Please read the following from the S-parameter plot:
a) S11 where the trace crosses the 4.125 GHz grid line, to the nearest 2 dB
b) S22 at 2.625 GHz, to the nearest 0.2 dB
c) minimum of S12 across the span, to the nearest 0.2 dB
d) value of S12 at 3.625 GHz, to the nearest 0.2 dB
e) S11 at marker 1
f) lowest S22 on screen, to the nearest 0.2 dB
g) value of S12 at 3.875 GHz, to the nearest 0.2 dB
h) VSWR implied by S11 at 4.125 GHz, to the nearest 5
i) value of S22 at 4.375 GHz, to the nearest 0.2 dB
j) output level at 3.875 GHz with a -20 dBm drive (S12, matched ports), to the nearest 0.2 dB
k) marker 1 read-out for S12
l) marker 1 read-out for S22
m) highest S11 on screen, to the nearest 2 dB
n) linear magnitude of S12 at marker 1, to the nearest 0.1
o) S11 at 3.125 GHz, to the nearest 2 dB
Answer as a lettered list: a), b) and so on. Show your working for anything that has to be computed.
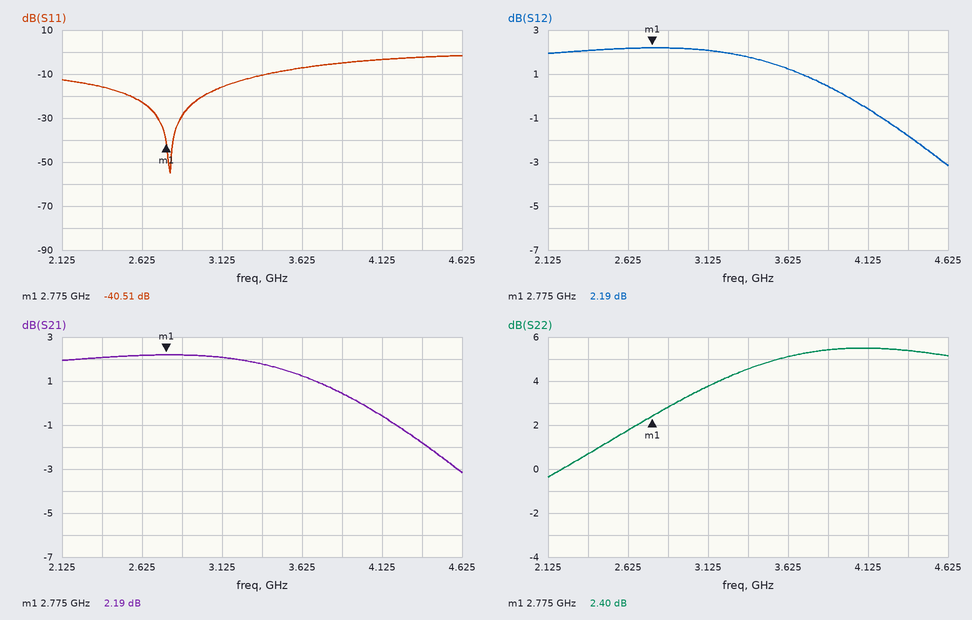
a) -4 dB
b) 1.8 dB
c) -3.2 dB
d) 1.2 dB
e) -40.51 dB
f) -0.4 dB
g) 0.4 dB
h) |Γ| = 10^(-4/20) = 0.6310; VSWR = (1 + 0.6310)/(1 − 0.6310) ≈ 4.42, so 5 to the nearest 5
i) 5.4 dB
j) -20 dBm + (0.4 dB) = -19.6 dBm
k) 2.19 dB
l) 2.40 dB
m) -2 dB
n) 10^(2.19/20) ≈ 1.3
o) -16 dB
